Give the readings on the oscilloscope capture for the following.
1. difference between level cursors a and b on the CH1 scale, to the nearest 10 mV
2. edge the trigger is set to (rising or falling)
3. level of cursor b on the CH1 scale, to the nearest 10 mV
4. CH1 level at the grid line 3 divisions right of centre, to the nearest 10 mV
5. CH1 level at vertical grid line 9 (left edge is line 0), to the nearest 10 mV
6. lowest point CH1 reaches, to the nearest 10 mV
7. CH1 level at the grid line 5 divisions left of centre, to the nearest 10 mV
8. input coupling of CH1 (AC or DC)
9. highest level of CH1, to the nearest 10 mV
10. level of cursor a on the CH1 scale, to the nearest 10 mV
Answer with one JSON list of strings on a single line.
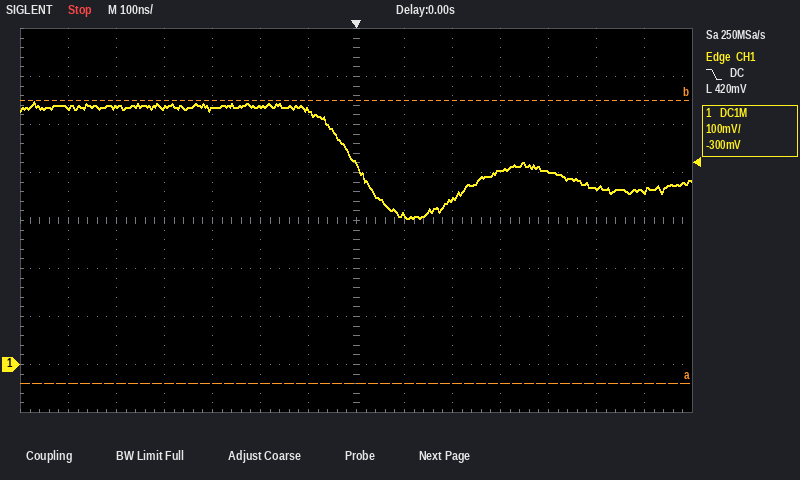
["590 mV", "falling", "550 mV", "400 mV", "340 mV", "300 mV", "540 mV", "DC", "550 mV", "-40 mV"]
